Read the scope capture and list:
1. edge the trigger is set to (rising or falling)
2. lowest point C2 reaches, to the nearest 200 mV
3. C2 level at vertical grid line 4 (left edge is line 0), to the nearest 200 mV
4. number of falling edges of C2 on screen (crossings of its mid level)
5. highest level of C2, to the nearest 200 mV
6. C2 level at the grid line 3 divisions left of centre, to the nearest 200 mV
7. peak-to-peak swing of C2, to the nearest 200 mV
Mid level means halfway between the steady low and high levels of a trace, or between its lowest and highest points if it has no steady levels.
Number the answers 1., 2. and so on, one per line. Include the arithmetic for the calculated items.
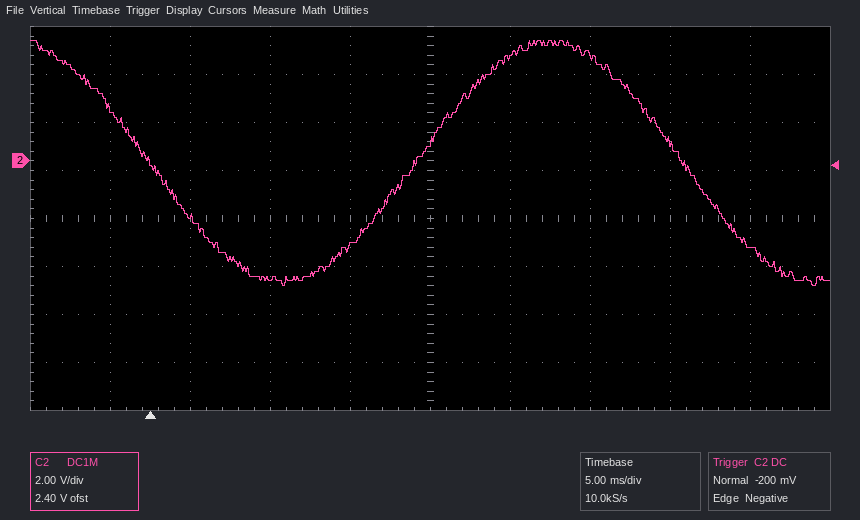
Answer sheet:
1. falling
2. -5.2 V
3. -3.6 V
4. 2
5. 5.0 V
6. -2.4 V
7. 5.0 V − (-5.2 V) = 10.2 V
